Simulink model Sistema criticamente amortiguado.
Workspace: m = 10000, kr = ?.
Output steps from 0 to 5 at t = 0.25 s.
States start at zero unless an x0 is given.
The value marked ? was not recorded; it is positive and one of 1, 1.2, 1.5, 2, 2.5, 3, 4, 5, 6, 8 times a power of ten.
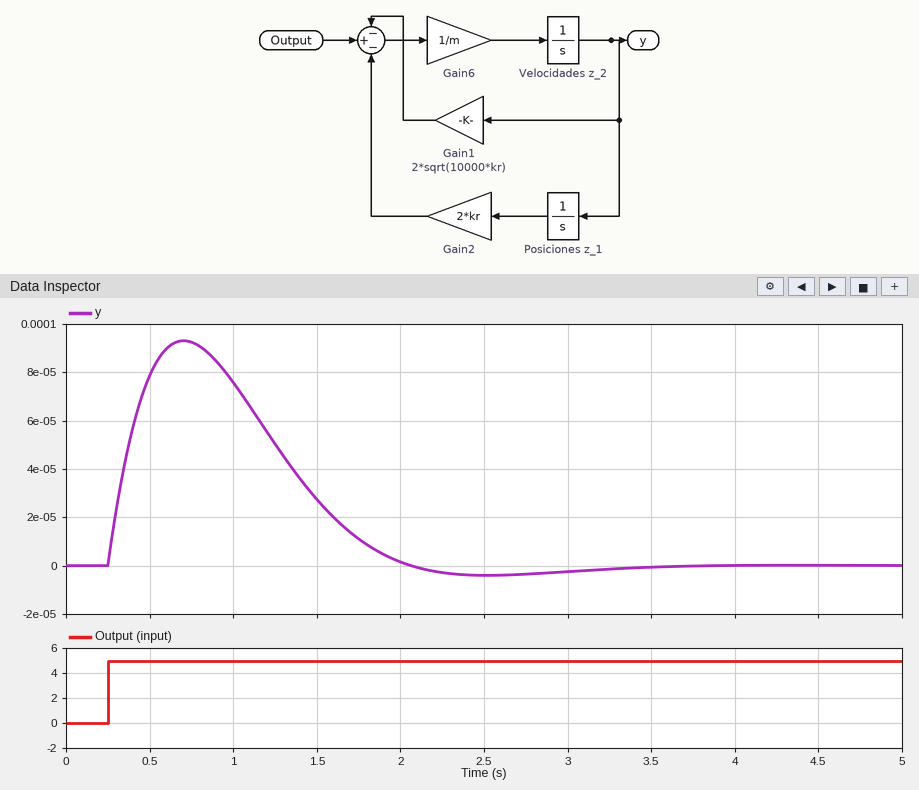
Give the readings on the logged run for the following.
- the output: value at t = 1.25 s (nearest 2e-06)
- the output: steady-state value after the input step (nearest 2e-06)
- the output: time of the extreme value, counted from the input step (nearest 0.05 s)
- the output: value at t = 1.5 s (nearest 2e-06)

0.000050
0.000000
0.45 s
0.000028
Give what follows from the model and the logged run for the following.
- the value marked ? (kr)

30000
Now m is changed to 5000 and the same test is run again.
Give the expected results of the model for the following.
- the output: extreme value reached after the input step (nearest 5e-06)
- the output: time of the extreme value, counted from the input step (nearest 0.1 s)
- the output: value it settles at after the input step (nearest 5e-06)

0.000105
0.3 s
0.000000
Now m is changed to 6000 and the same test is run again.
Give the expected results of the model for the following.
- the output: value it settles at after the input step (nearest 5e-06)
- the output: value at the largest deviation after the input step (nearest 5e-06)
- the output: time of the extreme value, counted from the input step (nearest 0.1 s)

0.000000
0.000105
0.3 s
